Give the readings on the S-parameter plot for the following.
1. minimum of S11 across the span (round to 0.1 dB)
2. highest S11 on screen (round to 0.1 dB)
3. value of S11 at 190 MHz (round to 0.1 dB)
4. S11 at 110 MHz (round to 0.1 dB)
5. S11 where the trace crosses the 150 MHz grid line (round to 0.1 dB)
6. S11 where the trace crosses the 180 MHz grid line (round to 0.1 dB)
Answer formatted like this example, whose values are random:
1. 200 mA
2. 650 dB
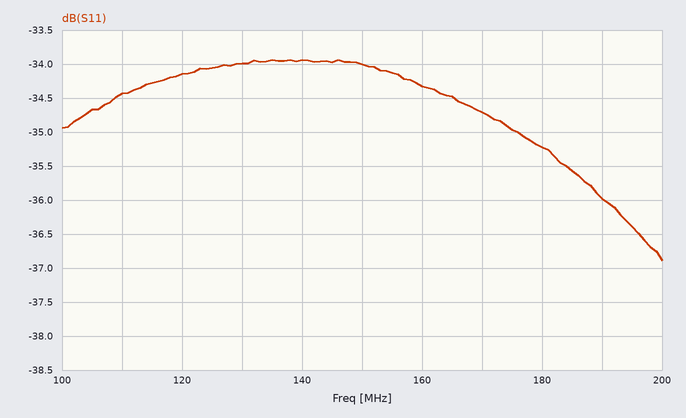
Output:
1. -36.9 dB
2. -33.9 dB
3. -36.0 dB
4. -34.4 dB
5. -34.0 dB
6. -35.2 dB
